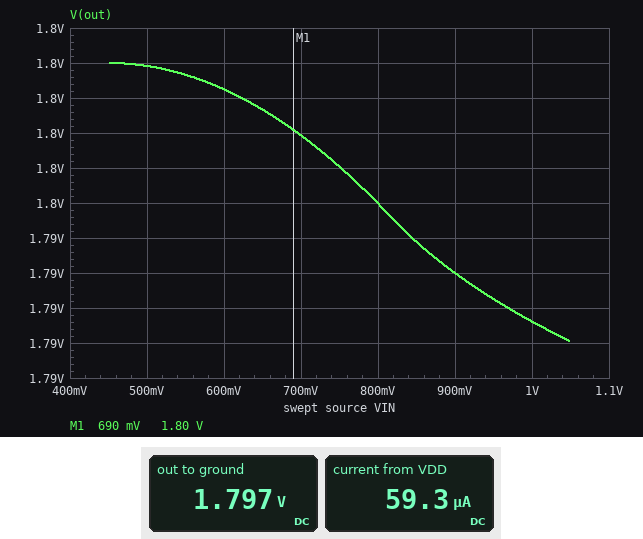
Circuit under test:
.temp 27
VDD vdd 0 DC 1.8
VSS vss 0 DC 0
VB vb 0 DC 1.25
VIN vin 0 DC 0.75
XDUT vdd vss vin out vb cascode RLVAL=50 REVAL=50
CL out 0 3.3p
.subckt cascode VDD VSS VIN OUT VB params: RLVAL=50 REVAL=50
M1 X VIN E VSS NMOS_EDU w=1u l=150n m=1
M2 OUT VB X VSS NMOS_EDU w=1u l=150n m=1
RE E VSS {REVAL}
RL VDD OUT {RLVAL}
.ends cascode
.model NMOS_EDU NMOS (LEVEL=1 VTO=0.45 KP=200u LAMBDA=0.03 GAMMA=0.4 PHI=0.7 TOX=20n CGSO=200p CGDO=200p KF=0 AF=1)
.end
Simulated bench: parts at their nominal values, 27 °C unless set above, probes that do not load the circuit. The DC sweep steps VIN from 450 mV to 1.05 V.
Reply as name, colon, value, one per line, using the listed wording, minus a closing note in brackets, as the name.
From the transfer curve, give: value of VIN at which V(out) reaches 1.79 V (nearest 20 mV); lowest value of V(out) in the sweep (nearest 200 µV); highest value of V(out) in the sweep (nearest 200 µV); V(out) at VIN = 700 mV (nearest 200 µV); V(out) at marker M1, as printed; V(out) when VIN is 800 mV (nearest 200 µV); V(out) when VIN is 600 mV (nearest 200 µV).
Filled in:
value of VIN at which V(out) reaches 1.79 V: 900 mV
lowest value of V(out) in the sweep: 1.7920 V
highest value of V(out) in the sweep: 1.8000 V
V(out) at VIN = 700 mV: 1.7980 V
V(out) at marker M1, as printed: 1.80 V
V(out) when VIN is 800 mV: 1.7960 V
V(out) when VIN is 600 mV: 1.7992 V
